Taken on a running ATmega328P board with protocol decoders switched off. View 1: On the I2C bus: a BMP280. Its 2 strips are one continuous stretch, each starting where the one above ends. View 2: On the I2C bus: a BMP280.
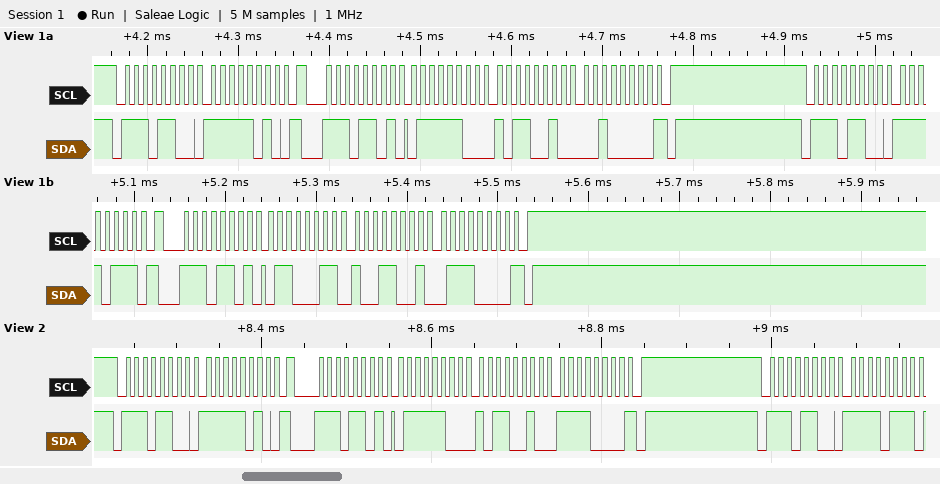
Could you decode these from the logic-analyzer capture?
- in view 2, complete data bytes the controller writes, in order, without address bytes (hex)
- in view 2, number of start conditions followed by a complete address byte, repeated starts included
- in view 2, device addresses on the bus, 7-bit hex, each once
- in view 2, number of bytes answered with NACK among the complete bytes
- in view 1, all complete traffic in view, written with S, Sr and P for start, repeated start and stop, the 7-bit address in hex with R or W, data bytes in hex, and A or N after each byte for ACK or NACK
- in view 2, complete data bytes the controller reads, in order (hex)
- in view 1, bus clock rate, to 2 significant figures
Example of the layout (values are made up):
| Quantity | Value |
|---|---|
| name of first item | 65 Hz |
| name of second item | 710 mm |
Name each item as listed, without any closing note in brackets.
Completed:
| Quantity | Value |
|---|---|
| in view 2, complete data bytes the controller writes, in order, without address bytes | FA F7 |
| in view 2, number of start conditions followed by a complete address byte, repeated starts included | 3 |
| in view 2, device addresses on the bus, 7-bit hex, each once | 0x76 |
| in view 2, number of bytes answered with NACK among the complete bytes | 1 |
| in view 1, all complete traffic in view, written with S, Sr and P for start, repeated start and stop, the 7-bit address in hex with R or W, data bytes in hex, and A or N after each byte for ACK or NACK | S 76W A FA A Sr 76R A 7C A B2 A 20 N P S 76W A F7 A Sr 76R A 63 A 99 A 70 N P |
| in view 2, complete data bytes the controller reads, in order | 7C B2 F0 |
| in view 1, bus clock rate, to 2 significant figures | 100 kHz |
